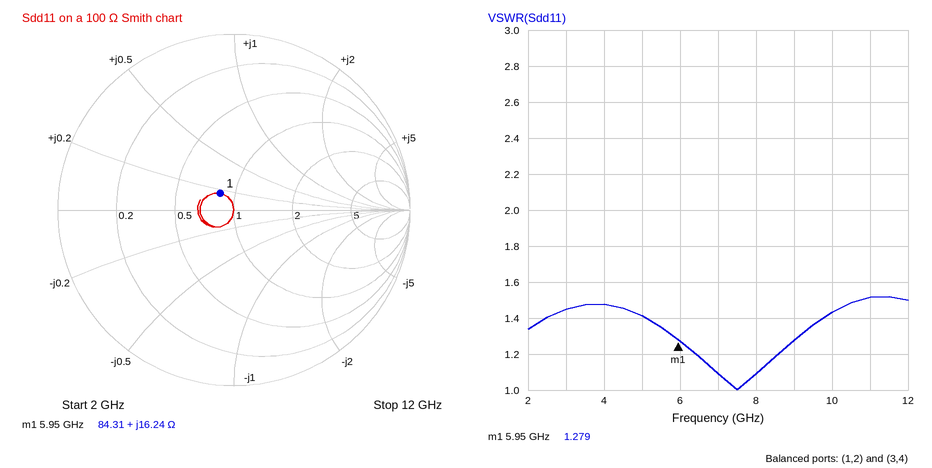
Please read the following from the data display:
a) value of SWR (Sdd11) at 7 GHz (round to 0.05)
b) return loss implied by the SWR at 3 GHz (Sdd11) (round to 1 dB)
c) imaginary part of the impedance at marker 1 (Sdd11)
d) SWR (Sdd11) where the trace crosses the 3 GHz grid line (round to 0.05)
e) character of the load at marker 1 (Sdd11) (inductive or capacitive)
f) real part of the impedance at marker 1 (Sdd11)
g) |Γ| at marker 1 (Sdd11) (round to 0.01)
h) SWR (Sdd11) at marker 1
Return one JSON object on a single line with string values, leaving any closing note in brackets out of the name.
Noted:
{"value of SWR (Sdd11) at 7 GHz": "1.10", "return loss implied by the SWR at 3 GHz (Sdd11)": "15 dB", "imaginary part of the impedance at marker 1": "+16.24 Ω", "SWR (Sdd11) where the trace crosses the 3 GHz grid line": "1.45", "character of the load at marker 1 (Sdd11)": "inductive", "real part of the impedance at marker 1": "84.31 Ω", "|Γ| at marker 1 (Sdd11)": "0.12", "SWR (Sdd11) at marker 1": "1.279"}
